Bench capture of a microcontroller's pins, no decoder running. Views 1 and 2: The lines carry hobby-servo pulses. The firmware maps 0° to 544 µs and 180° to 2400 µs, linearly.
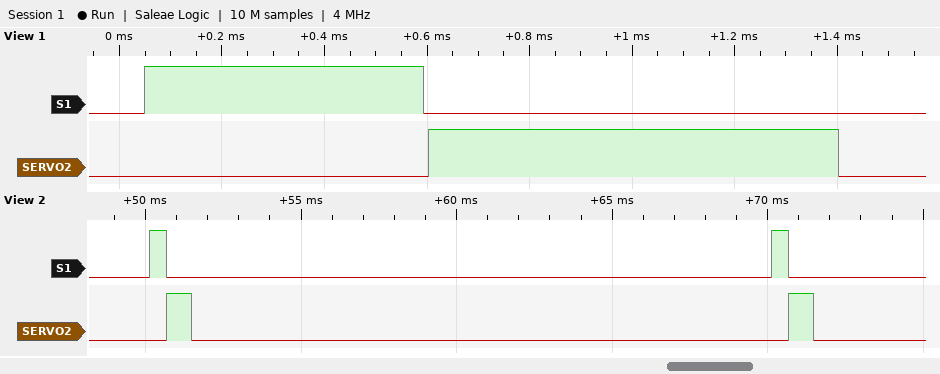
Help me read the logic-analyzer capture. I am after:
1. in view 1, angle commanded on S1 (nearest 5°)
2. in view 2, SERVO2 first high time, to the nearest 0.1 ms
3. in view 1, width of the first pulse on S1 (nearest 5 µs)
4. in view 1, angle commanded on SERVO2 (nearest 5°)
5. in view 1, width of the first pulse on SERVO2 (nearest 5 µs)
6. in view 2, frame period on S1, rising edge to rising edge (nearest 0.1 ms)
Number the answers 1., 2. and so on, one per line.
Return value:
1. 0°
2. 0.8 ms
3. 545 µs
4. 25°
5. 800 µs
6. 20.0 ms
